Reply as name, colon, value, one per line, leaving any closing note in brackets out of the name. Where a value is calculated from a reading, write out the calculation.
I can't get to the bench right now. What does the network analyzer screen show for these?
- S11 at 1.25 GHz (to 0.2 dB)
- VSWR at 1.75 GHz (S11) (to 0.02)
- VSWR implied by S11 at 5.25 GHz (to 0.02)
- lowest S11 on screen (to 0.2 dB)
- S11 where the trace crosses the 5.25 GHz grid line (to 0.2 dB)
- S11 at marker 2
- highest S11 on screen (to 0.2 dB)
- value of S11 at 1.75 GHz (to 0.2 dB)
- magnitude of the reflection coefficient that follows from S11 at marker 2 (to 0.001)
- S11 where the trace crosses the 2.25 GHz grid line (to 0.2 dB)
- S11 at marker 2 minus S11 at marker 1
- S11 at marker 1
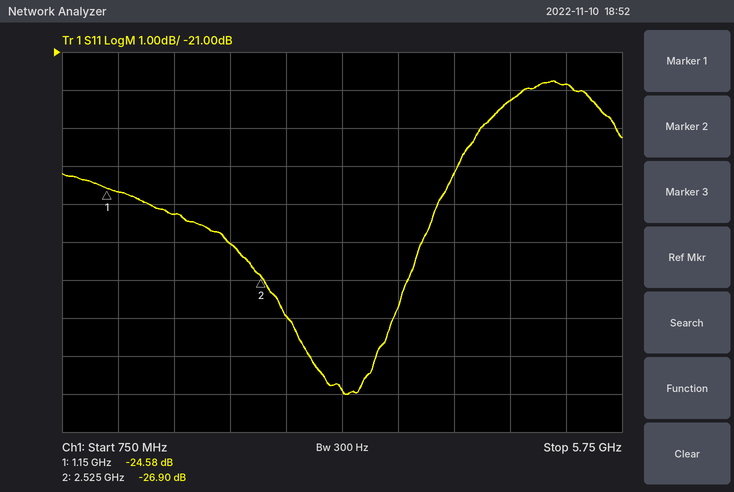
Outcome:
S11 at 1.25 GHz: -24.6 dB
VSWR at 1.75 GHz (S11): |Γ| = 10^(-25.2/20) = 0.0550; VSWR = (1 + 0.0550)/(1 − 0.0550) ≈ 1.12
VSWR implied by S11 at 5.25 GHz: |Γ| = 10^(-21.8/20) = 0.0813; VSWR = (1 + 0.0813)/(1 − 0.0813) ≈ 1.18
lowest S11 on screen: -30.0 dB
S11 where the trace crosses the 5.25 GHz grid line: -21.8 dB
S11 at marker 2: -26.90 dB
highest S11 on screen: -21.8 dB
value of S11 at 1.75 GHz: -25.2 dB
magnitude of the reflection coefficient that follows from S11 at marker 2: 10^(-26.9/20) ≈ 0.045
S11 where the trace crosses the 2.25 GHz grid line: -26.0 dB
S11 at marker 2 minus S11 at marker 1: -26.9 − (-24.58) = -2.32 dB
S11 at marker 1: -24.58 dB
